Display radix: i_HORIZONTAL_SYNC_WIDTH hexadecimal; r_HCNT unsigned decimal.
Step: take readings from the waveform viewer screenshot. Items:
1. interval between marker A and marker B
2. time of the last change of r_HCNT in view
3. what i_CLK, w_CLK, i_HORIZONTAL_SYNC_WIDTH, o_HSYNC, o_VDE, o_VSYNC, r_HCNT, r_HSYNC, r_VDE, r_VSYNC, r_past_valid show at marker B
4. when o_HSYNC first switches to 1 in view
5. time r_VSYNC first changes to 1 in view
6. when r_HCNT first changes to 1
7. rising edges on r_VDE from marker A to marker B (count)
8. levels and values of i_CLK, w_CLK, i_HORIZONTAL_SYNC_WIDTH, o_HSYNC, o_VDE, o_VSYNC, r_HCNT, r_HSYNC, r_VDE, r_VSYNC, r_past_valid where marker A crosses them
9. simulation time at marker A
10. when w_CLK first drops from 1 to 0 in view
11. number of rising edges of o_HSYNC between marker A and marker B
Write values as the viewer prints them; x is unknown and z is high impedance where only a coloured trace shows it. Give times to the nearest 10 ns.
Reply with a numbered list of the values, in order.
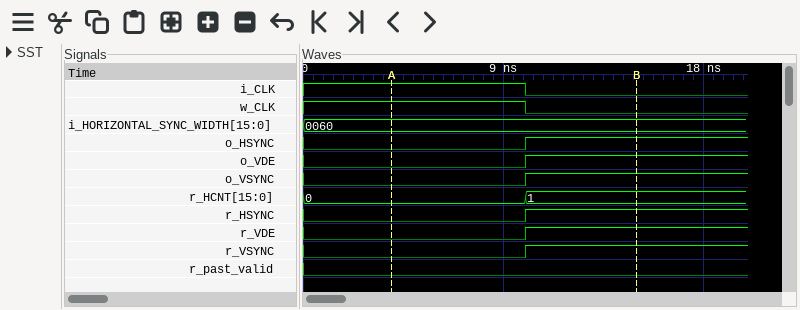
1. 10 ns
2. 10 ns
3. i_CLK=0, w_CLK=0, i_HORIZONTAL_SYNC_WIDTH=0060, o_HSYNC=1, o_VDE=1, o_VSYNC=1, r_HCNT=1, r_HSYNC=1, r_VDE=1, r_VSYNC=1, r_past_valid=0
4. 10 ns
5. 10 ns
6. 10 ns
7. 1
8. i_CLK=1, w_CLK=1, i_HORIZONTAL_SYNC_WIDTH=0060, o_HSYNC=0, o_VDE=0, o_VSYNC=0, r_HCNT=0, r_HSYNC=0, r_VDE=0, r_VSYNC=0, r_past_valid=0
9. 0 ns
10. 10 ns
11. 1
